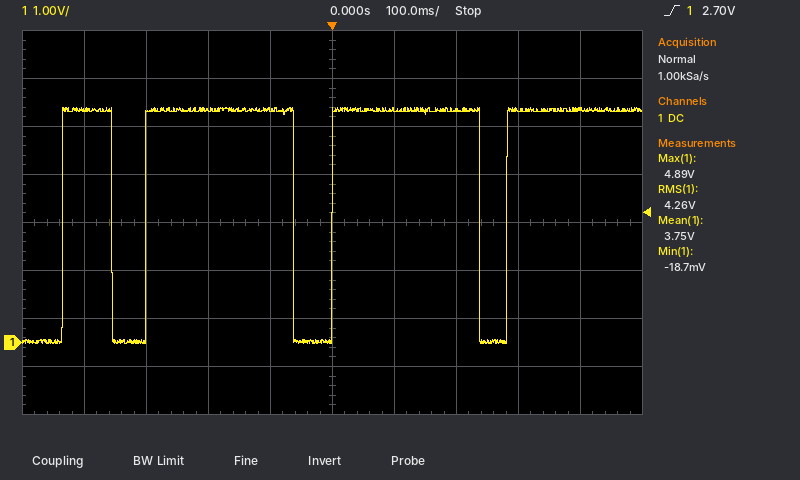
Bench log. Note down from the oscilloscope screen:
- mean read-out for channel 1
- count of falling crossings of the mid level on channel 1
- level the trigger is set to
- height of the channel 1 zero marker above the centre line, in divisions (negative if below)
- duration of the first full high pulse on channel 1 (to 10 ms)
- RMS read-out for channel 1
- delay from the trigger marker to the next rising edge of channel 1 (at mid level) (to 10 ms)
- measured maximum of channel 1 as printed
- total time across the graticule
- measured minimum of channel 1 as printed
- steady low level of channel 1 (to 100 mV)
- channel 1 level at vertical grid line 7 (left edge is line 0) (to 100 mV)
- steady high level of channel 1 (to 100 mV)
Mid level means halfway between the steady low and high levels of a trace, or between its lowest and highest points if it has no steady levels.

3.75 V
3
2.70 V
-2.5 div
80 ms
4.26 V
280 ms
4.89 V
1 s
-18.7 mV
0.0 V
4.8 V
4.8 V
